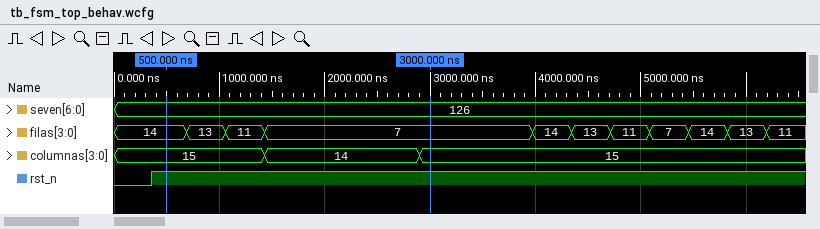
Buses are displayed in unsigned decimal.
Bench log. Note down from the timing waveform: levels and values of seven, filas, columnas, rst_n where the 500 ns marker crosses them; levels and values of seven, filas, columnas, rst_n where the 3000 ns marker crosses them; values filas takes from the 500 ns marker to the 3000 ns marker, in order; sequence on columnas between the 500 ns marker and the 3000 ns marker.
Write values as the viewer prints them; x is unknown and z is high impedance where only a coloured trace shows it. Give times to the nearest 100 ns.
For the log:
seven=126, filas=14, columnas=15, rst_n=1
seven=126, filas=7, columnas=15, rst_n=1
14, 13, 11, 7
15, 14, 15
